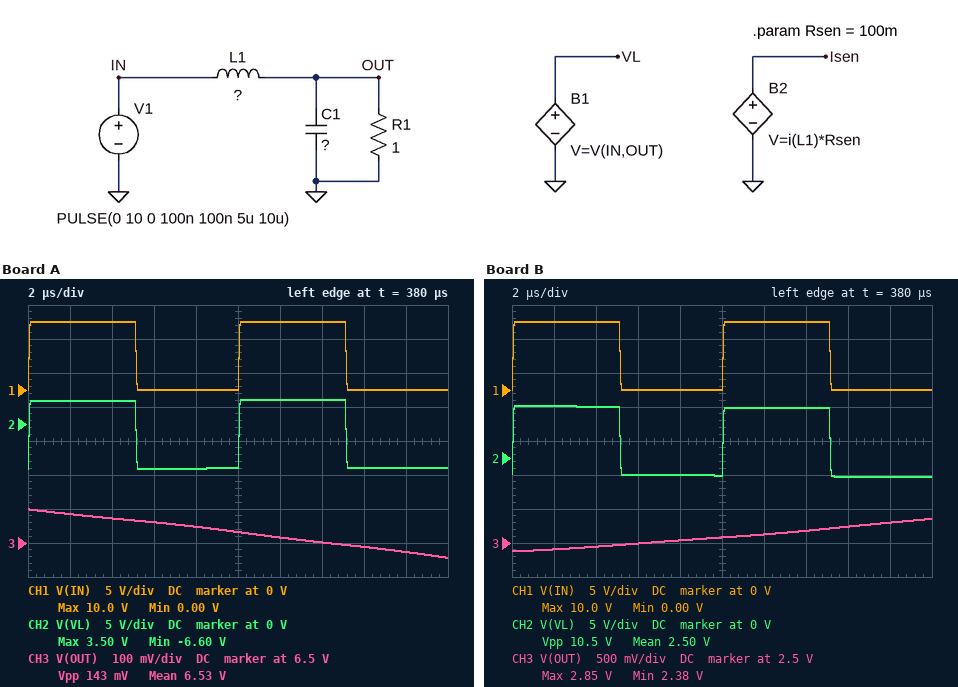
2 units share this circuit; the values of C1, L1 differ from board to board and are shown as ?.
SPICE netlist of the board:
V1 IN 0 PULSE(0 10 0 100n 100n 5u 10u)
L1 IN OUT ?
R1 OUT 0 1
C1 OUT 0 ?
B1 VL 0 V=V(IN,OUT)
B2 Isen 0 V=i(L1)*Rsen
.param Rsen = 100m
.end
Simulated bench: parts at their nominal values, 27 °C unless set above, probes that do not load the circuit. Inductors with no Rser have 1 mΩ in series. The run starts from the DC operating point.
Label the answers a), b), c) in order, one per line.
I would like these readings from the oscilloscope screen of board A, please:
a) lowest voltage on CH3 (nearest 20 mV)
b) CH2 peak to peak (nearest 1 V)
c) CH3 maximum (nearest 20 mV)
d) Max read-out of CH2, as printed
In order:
a) 6.46 V
b) 10 V
c) 6.60 V
d) 3.50 V
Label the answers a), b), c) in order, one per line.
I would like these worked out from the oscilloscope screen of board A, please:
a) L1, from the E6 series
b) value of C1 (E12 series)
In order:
a) 68 µH
b) 150 µF
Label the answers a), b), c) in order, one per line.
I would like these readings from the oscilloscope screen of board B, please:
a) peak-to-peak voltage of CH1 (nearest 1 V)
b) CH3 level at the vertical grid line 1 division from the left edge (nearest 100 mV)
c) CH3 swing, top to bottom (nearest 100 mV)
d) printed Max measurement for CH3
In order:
a) 10 V
b) 2.4 V
c) 500 mV
d) 2.85 V
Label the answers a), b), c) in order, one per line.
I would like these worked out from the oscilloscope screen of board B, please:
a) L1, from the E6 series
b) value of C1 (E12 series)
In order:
a) 10 µH
b) 330 µF
